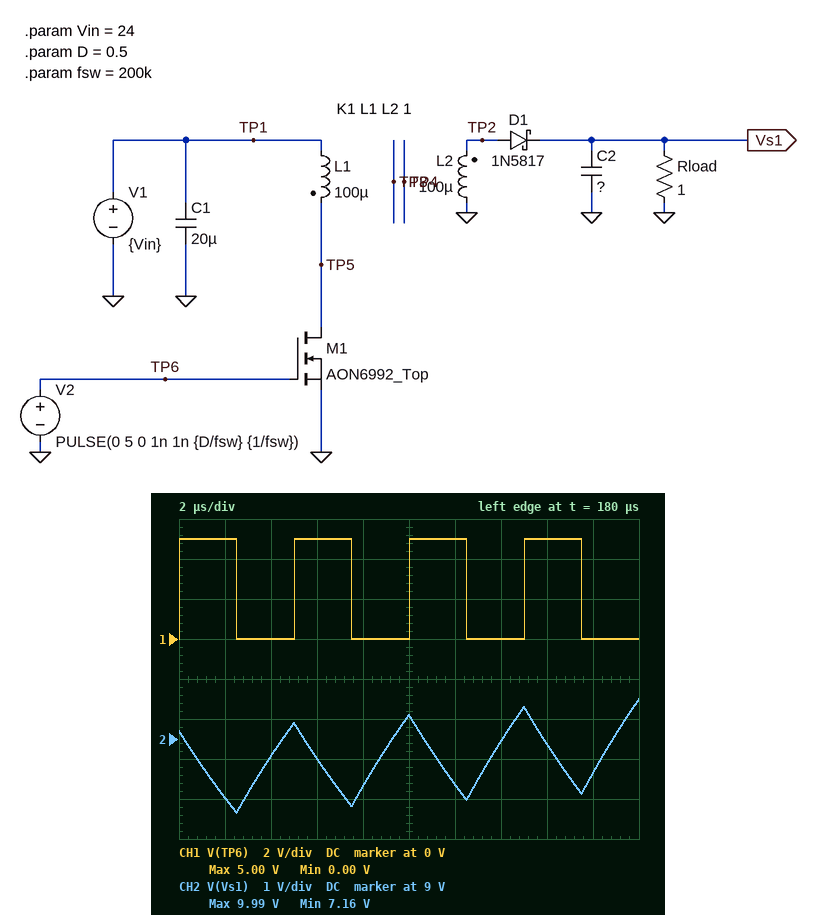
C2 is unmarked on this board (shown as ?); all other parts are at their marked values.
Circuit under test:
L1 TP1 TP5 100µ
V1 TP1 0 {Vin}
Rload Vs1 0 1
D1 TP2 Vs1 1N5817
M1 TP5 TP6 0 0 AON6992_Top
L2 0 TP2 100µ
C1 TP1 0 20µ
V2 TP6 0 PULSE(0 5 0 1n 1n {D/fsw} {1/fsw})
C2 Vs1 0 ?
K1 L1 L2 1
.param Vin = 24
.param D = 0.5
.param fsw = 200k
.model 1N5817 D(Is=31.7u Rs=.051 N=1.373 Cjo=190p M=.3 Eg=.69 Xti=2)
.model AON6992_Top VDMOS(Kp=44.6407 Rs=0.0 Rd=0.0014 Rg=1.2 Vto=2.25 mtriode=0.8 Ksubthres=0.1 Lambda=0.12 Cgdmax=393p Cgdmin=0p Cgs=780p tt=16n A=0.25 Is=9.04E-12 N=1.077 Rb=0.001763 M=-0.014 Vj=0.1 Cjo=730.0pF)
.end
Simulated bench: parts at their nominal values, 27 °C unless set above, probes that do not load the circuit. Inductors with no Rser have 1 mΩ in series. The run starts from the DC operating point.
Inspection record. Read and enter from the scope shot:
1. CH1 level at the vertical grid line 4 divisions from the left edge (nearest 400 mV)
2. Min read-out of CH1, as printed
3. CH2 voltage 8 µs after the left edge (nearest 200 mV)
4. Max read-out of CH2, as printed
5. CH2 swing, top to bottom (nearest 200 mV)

0 V
0.00 V
7.8 V
9.99 V
2.8 V
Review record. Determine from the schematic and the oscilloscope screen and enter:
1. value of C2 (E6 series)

10 µF
